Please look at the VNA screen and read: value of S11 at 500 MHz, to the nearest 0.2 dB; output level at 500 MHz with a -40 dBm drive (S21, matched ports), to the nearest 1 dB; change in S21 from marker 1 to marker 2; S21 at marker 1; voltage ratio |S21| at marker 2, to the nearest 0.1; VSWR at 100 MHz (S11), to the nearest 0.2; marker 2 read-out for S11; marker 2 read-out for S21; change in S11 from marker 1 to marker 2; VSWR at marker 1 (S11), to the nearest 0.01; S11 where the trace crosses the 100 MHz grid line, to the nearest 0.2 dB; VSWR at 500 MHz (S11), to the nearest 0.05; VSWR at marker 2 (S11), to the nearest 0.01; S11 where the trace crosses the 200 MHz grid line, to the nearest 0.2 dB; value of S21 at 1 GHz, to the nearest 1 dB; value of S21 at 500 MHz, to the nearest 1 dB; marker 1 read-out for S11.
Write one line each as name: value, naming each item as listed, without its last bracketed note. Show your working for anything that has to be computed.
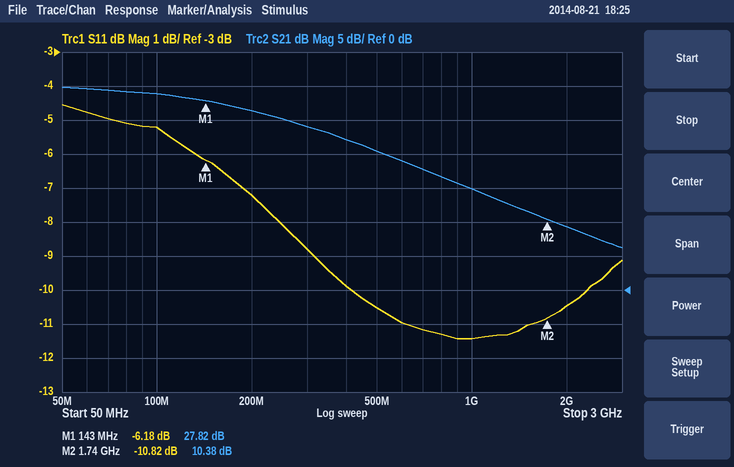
value of S11 at 500 MHz, to the nearest 0.2 dB: -10.6 dB
output level at 500 MHz with a -40 dBm drive (S21, matched ports), to the nearest 1 dB: -40 dBm + (20 dB) = -20 dBm
change in S21 from marker 1 to marker 2: 10.38 − (27.82) = -17.44 dB
S21 at marker 1: 27.82 dB
voltage ratio |S21| at marker 2, to the nearest 0.1: 10^(10.38/20) ≈ 3.3
VSWR at 100 MHz (S11), to the nearest 0.2: |Γ| = 10^(-5.2/20) = 0.5495; VSWR = (1 + 0.5495)/(1 − 0.5495) ≈ 3.4
marker 2 read-out for S11: -10.82 dB
marker 2 read-out for S21: 10.38 dB
change in S11 from marker 1 to marker 2: -10.82 − (-6.18) = -4.64 dB
VSWR at marker 1 (S11), to the nearest 0.01: (1 + 0.4909)/(1 − 0.4909) ≈ 2.93
S11 where the trace crosses the 100 MHz grid line, to the nearest 0.2 dB: -5.2 dB
VSWR at 500 MHz (S11), to the nearest 0.05: |Γ| = 10^(-10.6/20) = 0.2951; VSWR = (1 + 0.2951)/(1 − 0.2951) ≈ 1.84, so 1.85 to the nearest 0.05
VSWR at marker 2 (S11), to the nearest 0.01: (1 + 0.2877)/(1 − 0.2877) ≈ 1.81
S11 where the trace crosses the 200 MHz grid line, to the nearest 0.2 dB: -7.2 dB
value of S21 at 1 GHz, to the nearest 1 dB: 15 dB
value of S21 at 500 MHz, to the nearest 1 dB: 20 dB
marker 1 read-out for S11: -6.18 dB
